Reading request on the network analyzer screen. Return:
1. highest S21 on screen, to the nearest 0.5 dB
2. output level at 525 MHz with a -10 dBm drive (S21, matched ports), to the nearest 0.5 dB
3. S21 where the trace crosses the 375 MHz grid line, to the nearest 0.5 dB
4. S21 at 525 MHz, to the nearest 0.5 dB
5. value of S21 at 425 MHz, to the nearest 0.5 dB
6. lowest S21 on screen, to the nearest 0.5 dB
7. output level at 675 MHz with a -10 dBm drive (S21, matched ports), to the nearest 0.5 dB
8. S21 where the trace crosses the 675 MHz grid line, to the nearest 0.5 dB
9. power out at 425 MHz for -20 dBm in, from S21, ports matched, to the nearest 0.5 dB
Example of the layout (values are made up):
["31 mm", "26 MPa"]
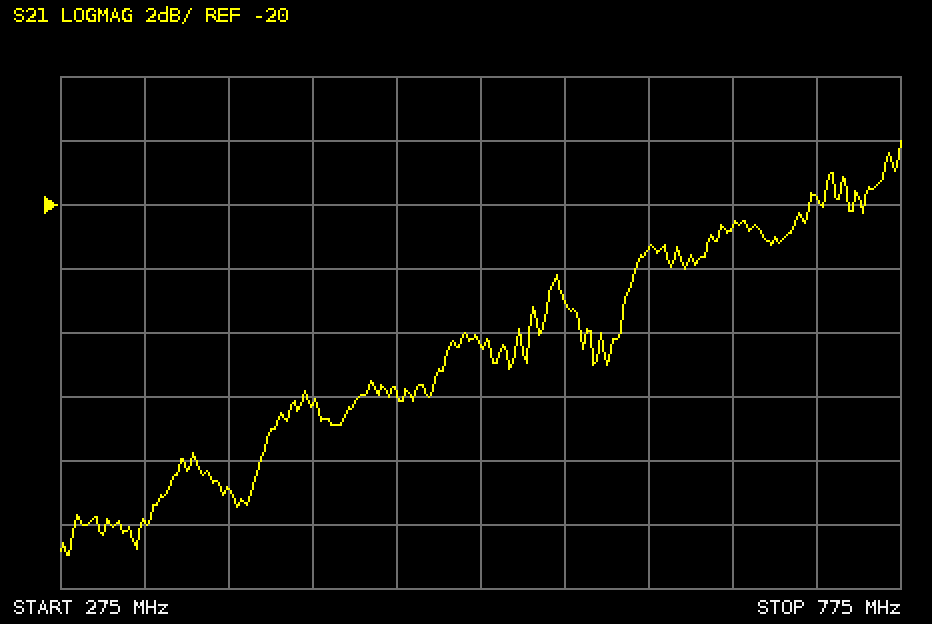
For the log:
["-18.0 dB", "-34.5 dBm", "-29.0 dB", "-24.5 dB", "-26.0 dB", "-31.0 dB", "-30.5 dBm", "-20.5 dB", "-46.0 dBm"]
